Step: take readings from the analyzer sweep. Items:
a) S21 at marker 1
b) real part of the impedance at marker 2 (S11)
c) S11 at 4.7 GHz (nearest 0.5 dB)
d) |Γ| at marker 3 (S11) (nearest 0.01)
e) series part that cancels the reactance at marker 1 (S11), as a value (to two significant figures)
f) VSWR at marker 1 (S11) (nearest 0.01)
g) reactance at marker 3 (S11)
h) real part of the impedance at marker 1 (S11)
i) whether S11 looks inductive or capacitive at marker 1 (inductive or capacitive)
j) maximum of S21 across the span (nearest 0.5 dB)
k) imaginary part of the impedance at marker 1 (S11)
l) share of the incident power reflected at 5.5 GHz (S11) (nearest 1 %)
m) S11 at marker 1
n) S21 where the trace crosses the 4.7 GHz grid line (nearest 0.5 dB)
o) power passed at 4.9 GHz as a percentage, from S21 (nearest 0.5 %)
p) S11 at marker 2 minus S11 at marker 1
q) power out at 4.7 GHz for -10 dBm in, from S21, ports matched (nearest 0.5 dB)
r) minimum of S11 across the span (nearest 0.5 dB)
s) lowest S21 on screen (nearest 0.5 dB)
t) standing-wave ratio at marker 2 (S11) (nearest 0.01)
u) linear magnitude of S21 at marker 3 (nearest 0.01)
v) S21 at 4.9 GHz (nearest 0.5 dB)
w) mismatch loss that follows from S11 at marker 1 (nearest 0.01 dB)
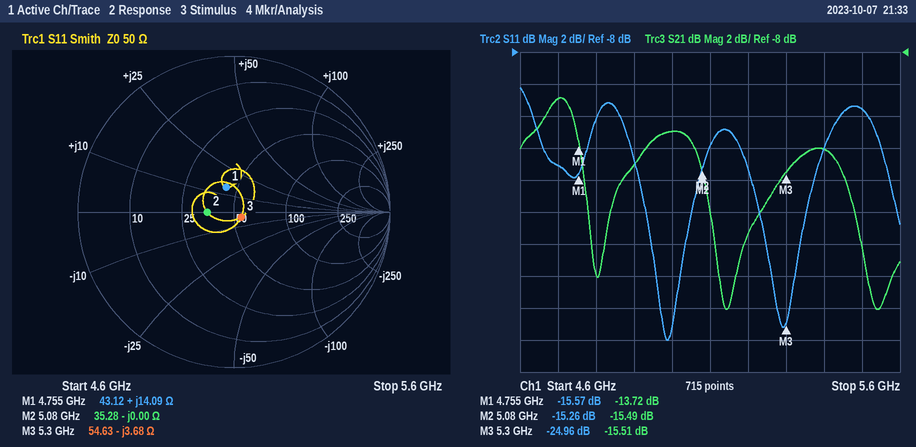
-13.72 dB
35.28 Ω
-15.0 dB
0.06
2.4 pF
1.40
-3.68 Ω
43.12 Ω
inductive
-11.0 dB
+14.09 Ω
7 %
-15.57 dB
-11.0 dB
3.0 %
0.31 dB
-21.0 dBm
-26.0 dB
-24.0 dB
1.42
0.17
-15.0 dB
0.12 dB
